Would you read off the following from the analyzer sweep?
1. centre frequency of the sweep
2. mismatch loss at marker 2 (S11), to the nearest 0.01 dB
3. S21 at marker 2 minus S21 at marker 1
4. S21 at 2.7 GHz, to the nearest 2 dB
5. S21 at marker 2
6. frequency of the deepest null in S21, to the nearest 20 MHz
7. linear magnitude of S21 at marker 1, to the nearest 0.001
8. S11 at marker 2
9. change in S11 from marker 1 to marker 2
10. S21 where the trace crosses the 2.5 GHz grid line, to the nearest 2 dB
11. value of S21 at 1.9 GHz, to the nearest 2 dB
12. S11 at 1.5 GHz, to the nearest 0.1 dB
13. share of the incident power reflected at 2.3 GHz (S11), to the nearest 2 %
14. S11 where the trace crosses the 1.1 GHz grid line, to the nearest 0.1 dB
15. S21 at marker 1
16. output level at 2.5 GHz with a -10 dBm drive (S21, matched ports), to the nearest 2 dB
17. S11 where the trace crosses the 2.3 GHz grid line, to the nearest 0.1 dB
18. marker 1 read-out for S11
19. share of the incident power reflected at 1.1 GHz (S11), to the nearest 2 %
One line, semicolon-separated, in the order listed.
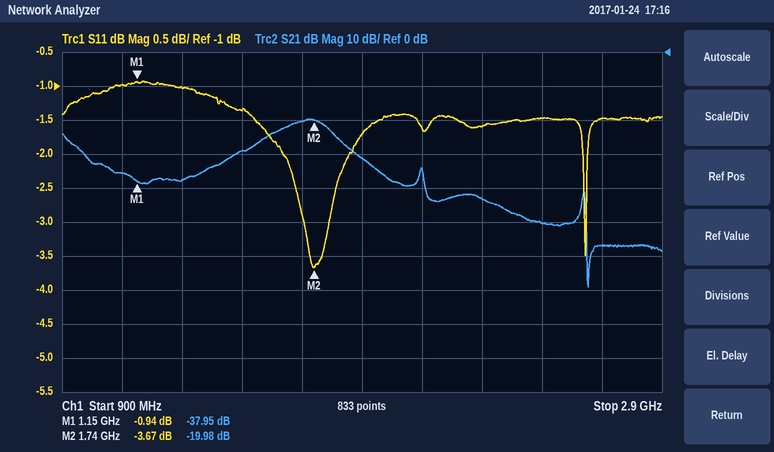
1.9 GHz; 2.44 dB; 17.97 dB; -56 dB; -19.98 dB; 2.66 GHz; 0.013; -3.67 dB; -2.73 dB; -50 dB; -32 dB; -1.4 dB; 70 %; -1.0 dB; -37.95 dB; -60 dBm; -1.6 dB; -0.94 dB; 80 %
